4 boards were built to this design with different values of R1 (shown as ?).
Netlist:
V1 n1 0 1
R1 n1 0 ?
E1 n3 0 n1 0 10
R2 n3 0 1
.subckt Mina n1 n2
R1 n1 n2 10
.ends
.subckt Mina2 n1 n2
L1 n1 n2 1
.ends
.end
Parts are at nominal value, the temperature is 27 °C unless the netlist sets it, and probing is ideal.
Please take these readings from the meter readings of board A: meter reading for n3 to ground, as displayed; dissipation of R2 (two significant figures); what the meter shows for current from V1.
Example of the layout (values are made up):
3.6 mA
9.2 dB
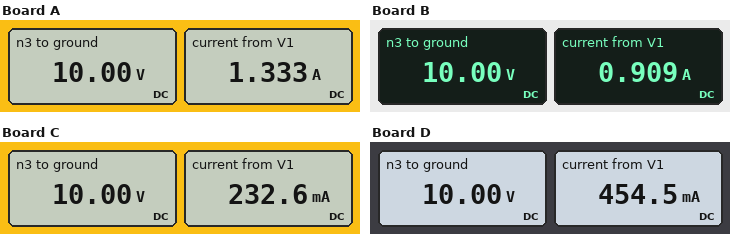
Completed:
10.00 V
100 W
1.333 A
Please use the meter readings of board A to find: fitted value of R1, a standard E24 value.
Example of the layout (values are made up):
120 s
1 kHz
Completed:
0.75 Ω
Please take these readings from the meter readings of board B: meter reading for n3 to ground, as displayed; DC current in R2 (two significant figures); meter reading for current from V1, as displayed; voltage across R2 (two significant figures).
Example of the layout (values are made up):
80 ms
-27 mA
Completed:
10.00 V
10 A
0.909 A
10 V
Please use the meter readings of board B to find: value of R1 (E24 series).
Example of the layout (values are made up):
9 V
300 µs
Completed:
1.1 Ω
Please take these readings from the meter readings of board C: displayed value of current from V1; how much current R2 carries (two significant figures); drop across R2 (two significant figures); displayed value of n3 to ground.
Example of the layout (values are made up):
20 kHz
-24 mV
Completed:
232.6 mA
10 A
10 V
10.00 V
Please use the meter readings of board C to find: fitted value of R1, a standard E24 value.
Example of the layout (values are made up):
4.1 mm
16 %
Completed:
4.3 Ω
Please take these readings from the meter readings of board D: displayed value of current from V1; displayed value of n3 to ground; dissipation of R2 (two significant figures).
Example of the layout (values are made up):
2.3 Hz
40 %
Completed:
454.5 mA
10.00 V
100 W
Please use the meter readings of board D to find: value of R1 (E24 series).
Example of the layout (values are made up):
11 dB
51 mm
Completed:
2.2 Ω
